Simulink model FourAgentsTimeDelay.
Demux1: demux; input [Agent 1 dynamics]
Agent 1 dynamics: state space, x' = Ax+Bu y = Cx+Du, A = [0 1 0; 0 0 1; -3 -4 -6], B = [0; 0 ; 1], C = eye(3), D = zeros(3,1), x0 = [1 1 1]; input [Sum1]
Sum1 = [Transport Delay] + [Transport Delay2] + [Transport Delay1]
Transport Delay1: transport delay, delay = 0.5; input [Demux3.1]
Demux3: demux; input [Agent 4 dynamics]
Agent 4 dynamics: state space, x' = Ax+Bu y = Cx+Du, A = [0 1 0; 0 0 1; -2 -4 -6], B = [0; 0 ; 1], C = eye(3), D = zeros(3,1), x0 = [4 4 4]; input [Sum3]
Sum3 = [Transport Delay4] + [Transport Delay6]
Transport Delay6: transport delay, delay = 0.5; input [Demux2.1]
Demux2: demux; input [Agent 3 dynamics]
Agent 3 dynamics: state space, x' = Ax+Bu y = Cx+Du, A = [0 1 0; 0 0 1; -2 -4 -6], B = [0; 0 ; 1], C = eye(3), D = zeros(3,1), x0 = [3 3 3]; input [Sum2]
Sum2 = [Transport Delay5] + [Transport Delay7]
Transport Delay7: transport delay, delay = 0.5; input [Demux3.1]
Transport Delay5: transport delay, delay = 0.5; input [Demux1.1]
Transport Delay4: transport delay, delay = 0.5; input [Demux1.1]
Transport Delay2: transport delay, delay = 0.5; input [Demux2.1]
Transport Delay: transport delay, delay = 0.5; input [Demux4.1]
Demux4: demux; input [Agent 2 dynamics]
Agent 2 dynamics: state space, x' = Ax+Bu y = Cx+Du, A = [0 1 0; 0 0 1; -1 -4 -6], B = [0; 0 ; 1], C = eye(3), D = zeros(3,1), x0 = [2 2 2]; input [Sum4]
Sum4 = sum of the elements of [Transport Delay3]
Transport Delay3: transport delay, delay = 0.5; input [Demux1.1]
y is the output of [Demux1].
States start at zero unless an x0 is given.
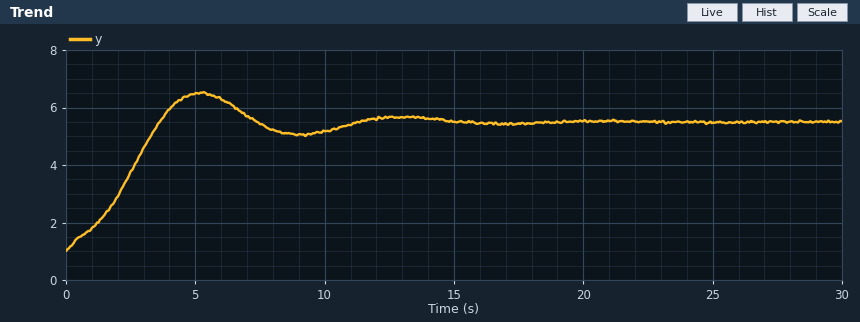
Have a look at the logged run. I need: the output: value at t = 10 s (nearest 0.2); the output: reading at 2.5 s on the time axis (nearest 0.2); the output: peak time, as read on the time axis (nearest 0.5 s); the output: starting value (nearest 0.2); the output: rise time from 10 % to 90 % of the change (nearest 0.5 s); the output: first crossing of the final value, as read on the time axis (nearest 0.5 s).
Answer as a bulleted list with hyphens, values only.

- 5.2
- 3.8
- 5.0 s
- 1.0
- 3.0 s
- 3.5 s
